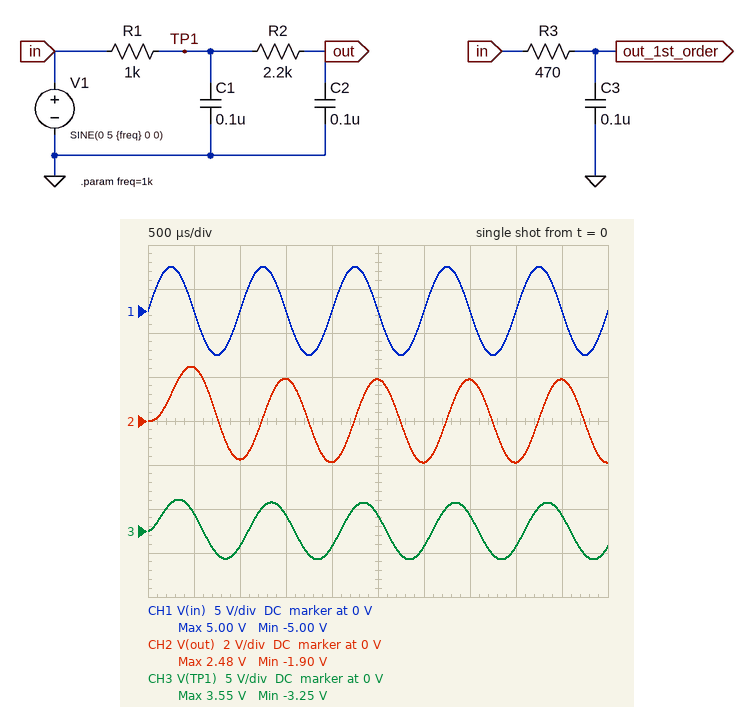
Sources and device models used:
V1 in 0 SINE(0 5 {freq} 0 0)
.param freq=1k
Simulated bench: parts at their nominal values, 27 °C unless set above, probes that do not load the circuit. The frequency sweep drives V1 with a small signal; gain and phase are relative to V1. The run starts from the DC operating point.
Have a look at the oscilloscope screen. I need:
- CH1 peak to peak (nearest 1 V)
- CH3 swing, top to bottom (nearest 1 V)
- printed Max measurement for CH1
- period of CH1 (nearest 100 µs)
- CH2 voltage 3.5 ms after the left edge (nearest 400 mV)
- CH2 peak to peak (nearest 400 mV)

10 V
7 V
5.00 V
1.0 ms
2.0 V
4.4 V
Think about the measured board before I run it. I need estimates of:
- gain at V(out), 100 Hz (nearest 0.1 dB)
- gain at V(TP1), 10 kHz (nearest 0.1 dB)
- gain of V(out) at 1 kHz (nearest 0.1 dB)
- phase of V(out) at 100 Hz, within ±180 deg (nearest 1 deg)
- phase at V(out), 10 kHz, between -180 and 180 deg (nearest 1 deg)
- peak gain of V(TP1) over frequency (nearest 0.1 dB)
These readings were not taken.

-0.2 dB
-16.2 dB
-8.4 dB
-15 deg
-163 deg
0 dB
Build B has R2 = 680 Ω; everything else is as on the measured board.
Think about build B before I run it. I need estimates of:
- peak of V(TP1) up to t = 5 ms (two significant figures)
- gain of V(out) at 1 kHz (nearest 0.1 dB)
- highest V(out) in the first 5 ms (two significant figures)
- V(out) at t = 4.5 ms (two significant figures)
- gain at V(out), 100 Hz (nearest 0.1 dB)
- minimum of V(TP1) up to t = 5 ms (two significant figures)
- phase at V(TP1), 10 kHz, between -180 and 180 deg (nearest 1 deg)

3.4 V
-5.3 dB
3.2 V
2.5 V
-0.1 dB
-3.0 V
-70 deg
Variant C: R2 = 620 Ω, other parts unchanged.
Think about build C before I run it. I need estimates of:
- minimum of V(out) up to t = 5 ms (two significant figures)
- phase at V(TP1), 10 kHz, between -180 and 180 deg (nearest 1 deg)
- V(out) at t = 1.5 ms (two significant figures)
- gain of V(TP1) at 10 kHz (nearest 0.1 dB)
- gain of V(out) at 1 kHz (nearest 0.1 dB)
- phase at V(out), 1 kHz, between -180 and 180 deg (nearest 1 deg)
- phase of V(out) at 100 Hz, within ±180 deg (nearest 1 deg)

-2.8 V
-69 deg
2.5 V
-17.1 dB
-5.2 dB
-65 deg
-9 deg
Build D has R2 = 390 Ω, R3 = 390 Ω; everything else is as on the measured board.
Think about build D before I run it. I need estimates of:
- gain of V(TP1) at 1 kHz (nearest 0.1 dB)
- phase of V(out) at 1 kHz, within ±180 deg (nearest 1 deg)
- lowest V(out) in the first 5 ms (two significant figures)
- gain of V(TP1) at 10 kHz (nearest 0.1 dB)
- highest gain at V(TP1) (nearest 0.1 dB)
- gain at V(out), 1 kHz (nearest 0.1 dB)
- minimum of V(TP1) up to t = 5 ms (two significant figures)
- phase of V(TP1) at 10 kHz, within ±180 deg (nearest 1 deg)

-4.5 dB
-61 deg
-2.9 V
-17.9 dB
0 dB
-4.7 dB
-3.0 V
-66 deg
